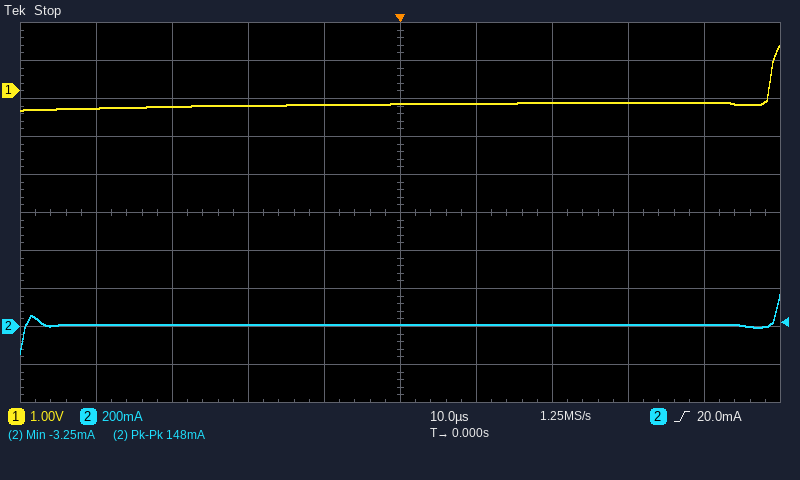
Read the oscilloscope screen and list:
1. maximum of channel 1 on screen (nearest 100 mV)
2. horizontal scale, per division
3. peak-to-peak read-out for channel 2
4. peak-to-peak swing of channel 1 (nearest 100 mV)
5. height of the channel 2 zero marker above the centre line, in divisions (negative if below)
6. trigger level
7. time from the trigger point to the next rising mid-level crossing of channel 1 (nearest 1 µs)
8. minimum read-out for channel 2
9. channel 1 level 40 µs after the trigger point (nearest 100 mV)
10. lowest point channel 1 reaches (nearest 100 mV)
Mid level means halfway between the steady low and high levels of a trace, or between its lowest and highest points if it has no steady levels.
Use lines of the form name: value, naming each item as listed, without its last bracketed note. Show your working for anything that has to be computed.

maximum of channel 1 on screen: 1.2 V
horizontal scale, per division: 10 µs
peak-to-peak read-out for channel 2: 148 mA
peak-to-peak swing of channel 1: 1.2 V − (-500 mV) = 1.7 V
height of the channel 2 zero marker above the centre line, in divisions: -3.0 div
trigger level: 20.0 mA
time from the trigger point to the next rising mid-level crossing of channel 1: 49 µs
minimum read-out for channel 2: -3.25 mA
channel 1 level 40 µs after the trigger point: -300 mV
lowest point channel 1 reaches: -500 mV
